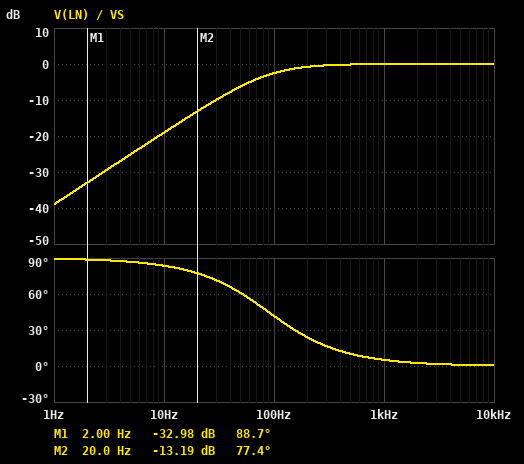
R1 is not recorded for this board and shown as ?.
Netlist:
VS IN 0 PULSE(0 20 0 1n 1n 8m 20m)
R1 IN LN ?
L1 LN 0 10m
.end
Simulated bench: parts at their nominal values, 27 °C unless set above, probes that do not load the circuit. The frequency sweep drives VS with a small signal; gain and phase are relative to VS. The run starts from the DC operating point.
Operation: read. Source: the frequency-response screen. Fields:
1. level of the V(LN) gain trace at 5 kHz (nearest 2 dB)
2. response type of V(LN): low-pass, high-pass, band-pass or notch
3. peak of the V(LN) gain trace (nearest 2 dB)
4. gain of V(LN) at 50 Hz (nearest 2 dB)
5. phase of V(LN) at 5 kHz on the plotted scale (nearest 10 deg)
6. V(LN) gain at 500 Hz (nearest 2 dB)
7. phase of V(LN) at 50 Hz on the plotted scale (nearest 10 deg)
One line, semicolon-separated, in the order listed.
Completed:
0 dB; high-pass; 0 dB; -6 dB; 0 deg; 0 dB; 60 deg
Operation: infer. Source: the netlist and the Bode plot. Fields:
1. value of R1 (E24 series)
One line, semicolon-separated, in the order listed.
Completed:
5.6 Ω
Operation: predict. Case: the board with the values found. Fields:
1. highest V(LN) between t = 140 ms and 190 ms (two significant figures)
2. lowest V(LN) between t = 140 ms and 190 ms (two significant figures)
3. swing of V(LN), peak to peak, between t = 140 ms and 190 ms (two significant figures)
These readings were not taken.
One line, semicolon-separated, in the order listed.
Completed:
20 V; -20 V; 40 V
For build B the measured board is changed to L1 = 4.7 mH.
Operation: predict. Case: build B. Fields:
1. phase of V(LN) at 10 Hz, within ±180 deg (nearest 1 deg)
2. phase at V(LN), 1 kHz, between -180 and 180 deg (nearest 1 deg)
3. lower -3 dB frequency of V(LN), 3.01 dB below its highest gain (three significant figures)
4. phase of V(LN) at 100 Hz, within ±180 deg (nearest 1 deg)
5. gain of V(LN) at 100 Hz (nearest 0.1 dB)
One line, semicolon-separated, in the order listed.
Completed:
87 deg; 11 deg; 190 Hz; 62 deg; -6.6 dB
